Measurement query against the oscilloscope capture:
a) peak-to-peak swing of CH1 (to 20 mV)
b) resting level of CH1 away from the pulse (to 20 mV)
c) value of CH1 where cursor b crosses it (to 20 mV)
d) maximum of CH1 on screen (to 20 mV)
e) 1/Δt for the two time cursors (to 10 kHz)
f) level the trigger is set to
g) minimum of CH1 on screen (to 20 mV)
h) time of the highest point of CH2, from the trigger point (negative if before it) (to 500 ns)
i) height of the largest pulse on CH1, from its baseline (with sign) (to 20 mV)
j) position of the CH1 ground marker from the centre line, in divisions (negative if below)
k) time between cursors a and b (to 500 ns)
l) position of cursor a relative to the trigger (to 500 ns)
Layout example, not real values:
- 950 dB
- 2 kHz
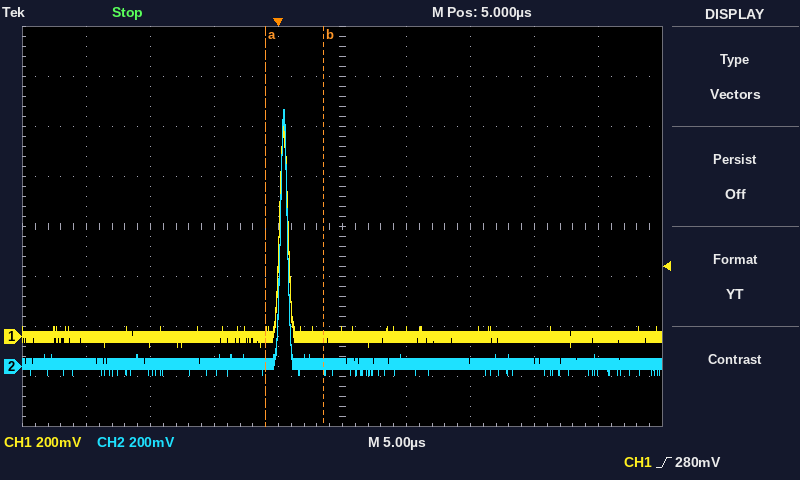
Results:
- 880 mV
- 0 mV
- 0 mV
- 840 mV
- 220 kHz
- 280 mV
- -40 mV
- +500 ns
- +840 mV
- -2.2 div
- 4.5 µs
- -1.0 µs
